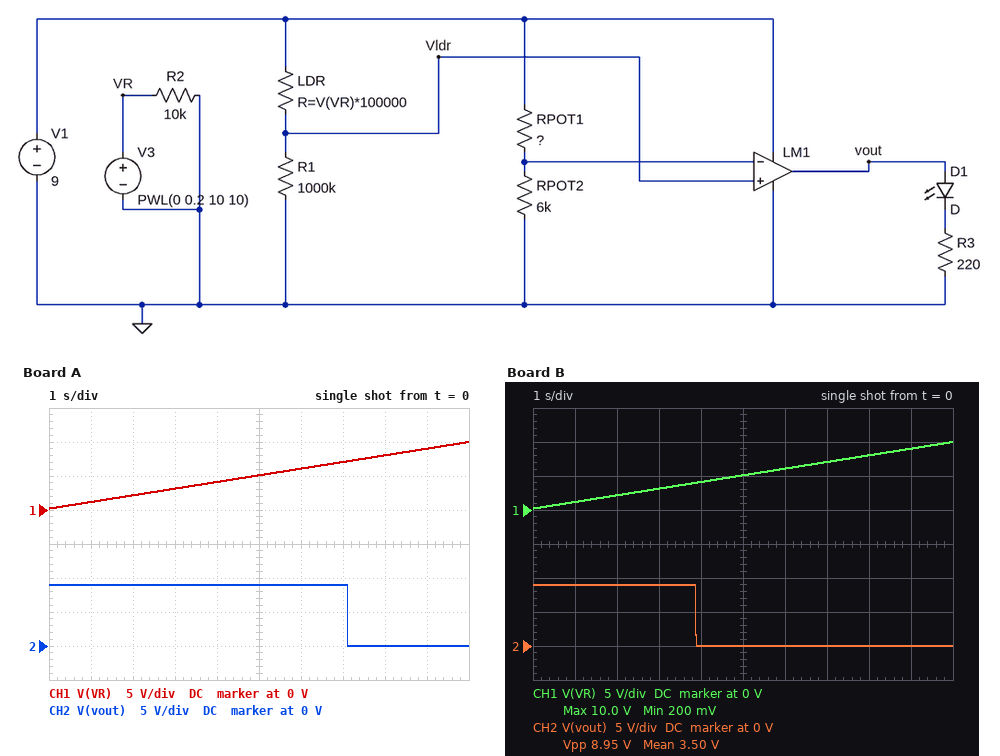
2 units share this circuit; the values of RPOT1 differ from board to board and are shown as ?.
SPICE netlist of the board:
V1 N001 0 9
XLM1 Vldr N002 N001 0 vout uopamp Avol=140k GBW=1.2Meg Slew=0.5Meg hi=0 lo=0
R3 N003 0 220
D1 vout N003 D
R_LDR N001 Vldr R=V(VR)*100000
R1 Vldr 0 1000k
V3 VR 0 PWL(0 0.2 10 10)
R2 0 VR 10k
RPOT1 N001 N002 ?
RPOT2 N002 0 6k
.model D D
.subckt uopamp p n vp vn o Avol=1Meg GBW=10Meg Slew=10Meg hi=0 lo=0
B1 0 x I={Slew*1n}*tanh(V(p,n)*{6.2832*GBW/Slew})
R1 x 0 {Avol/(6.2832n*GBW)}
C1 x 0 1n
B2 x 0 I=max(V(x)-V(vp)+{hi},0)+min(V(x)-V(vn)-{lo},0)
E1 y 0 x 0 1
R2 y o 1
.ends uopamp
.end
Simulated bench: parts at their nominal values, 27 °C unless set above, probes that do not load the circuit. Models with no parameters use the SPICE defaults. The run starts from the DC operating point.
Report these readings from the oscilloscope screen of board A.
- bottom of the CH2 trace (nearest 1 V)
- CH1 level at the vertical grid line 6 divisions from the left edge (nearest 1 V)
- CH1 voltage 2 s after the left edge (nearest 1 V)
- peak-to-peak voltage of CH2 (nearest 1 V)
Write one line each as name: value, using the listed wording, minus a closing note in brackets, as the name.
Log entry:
bottom of the CH2 trace: 0 V
CH1 level at the vertical grid line 6 divisions from the left edge: 6 V
CH1 voltage 2 s after the left edge: 2 V
peak-to-peak voltage of CH2: 9 V
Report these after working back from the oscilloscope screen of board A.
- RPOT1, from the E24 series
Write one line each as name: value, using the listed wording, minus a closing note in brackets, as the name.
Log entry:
RPOT1, from the E24 series: 4.3 kΩ
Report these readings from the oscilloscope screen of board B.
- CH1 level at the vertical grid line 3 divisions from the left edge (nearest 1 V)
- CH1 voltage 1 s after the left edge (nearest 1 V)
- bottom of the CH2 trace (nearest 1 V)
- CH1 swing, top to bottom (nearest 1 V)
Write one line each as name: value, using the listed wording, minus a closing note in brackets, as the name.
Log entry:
CH1 level at the vertical grid line 3 divisions from the left edge: 3 V
CH1 voltage 1 s after the left edge: 1 V
bottom of the CH2 trace: 0 V
CH1 swing, top to bottom: 10 V
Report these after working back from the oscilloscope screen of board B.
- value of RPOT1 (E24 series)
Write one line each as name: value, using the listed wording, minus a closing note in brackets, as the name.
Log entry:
value of RPOT1: 2.4 kΩ
